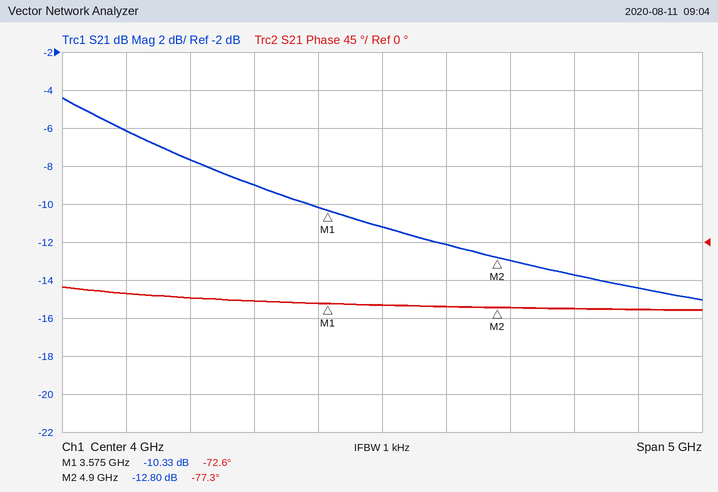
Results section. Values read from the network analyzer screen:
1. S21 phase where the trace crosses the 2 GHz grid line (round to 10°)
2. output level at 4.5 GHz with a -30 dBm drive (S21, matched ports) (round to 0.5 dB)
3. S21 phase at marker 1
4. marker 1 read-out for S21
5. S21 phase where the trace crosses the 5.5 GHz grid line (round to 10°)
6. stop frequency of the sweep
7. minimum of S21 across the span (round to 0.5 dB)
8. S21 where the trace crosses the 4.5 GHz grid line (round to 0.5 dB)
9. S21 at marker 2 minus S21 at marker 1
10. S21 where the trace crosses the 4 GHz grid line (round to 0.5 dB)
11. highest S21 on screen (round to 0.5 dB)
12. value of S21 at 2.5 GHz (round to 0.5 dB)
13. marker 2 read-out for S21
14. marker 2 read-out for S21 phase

-60°
-42.0 dBm
-72.6°
-10.33 dB
-80°
6.5 GHz
-15.0 dB
-12.0 dB
-2.47 dB
-11.0 dB
-4.5 dB
-7.5 dB
-12.80 dB
-77.3°
